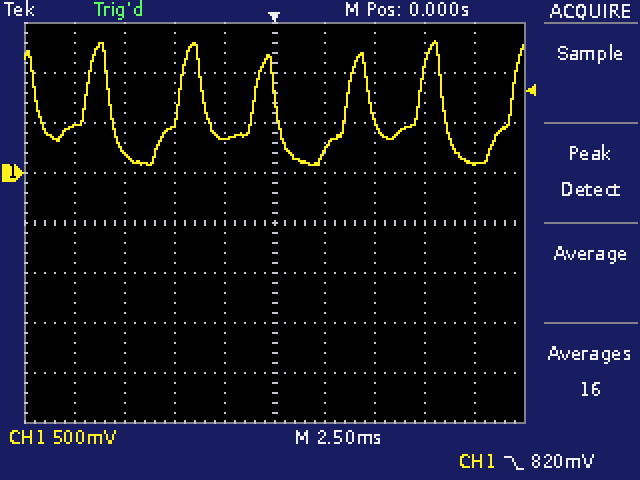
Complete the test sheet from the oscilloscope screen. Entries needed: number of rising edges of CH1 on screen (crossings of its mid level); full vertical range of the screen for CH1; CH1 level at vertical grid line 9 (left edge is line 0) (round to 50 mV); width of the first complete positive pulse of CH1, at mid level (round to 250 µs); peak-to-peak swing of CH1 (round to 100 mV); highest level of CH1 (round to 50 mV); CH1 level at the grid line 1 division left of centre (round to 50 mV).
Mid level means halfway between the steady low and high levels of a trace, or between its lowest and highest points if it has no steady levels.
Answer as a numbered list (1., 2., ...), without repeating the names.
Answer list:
1. 6
2. 4 V
3. 100 mV
4. 1.25 ms
5. 1.20 V
6. 1.30 V
7. 350 mV
